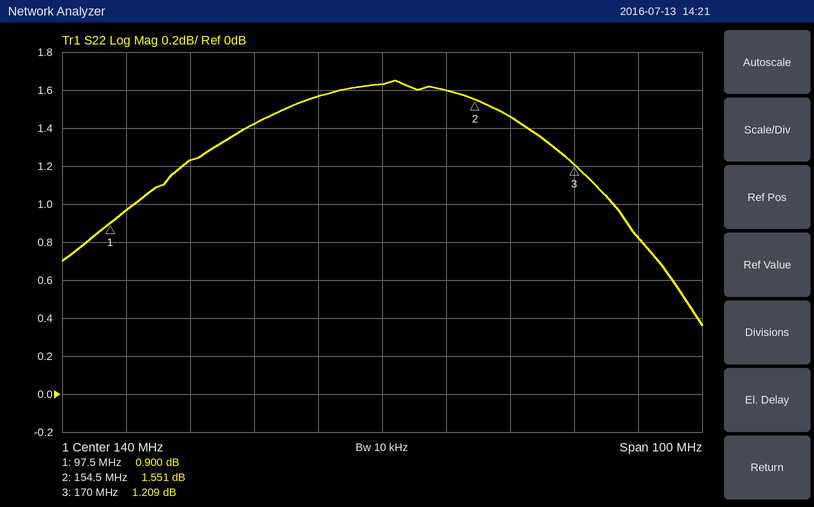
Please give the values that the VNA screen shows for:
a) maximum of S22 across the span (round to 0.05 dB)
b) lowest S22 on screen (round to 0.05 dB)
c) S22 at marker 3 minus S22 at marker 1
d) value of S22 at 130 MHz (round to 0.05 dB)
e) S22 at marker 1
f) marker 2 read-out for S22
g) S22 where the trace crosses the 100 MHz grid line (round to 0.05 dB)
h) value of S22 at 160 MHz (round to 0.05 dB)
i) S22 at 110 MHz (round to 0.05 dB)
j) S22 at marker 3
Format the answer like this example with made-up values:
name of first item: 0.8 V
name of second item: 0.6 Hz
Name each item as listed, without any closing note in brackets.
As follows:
maximum of S22 across the span: 1.65 dB
lowest S22 on screen: 0.35 dB
S22 at marker 3 minus S22 at marker 1: 0.309 dB
value of S22 at 130 MHz: 1.55 dB
S22 at marker 1: 0.900 dB
marker 2 read-out for S22: 1.551 dB
S22 where the trace crosses the 100 MHz grid line: 0.95 dB
value of S22 at 160 MHz: 1.45 dB
S22 at 110 MHz: 1.25 dB
S22 at marker 3: 1.209 dB
